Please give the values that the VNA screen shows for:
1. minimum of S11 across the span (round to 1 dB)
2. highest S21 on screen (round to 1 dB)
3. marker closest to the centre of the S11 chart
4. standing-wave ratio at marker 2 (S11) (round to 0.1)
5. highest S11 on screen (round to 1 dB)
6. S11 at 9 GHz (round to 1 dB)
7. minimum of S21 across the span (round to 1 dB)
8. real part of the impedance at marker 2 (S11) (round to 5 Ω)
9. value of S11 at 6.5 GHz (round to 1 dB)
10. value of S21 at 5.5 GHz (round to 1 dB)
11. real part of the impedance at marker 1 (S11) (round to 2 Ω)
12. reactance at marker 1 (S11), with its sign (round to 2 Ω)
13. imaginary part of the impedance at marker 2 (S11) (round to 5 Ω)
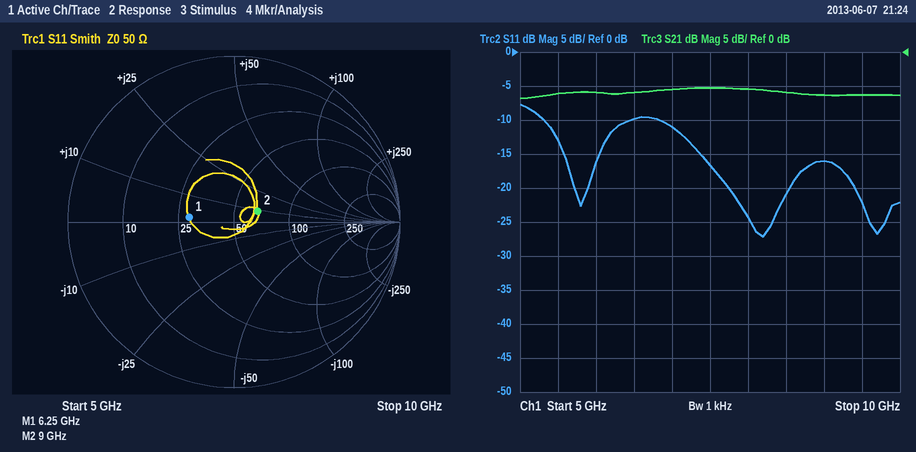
-27 dB
-5 dB
marker 2
1.4
-8 dB
-16 dB
-7 dB
65 Ω
-10 dB
-6 dB
28 Ω
+2 Ω
+10 Ω
